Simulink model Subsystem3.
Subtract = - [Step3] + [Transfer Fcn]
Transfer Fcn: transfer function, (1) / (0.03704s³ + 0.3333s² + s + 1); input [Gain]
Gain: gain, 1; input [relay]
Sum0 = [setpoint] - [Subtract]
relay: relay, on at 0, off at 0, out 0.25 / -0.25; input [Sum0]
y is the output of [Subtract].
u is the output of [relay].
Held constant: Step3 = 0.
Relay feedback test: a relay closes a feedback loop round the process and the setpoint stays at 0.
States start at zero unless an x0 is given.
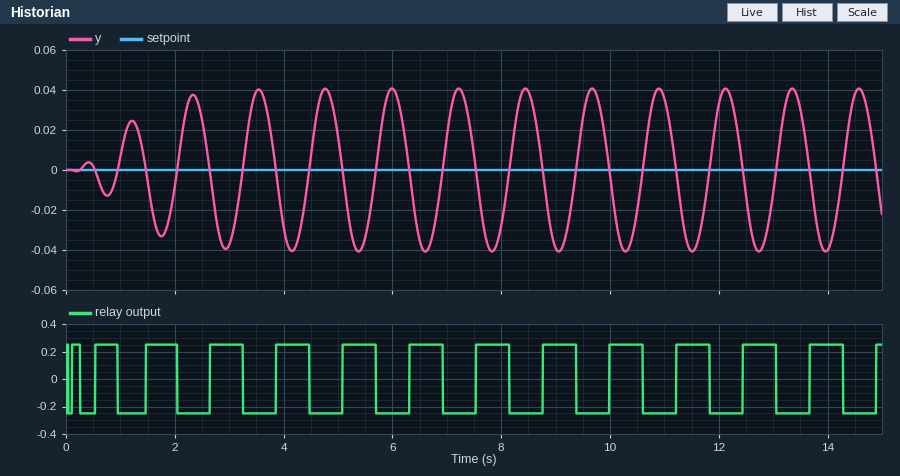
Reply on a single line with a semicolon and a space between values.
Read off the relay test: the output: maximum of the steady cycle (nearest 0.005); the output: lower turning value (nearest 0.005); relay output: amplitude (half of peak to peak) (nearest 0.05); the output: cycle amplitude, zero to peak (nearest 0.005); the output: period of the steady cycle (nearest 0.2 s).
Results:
0.040; -0.040; 0.25; 0.040; 1.2 s
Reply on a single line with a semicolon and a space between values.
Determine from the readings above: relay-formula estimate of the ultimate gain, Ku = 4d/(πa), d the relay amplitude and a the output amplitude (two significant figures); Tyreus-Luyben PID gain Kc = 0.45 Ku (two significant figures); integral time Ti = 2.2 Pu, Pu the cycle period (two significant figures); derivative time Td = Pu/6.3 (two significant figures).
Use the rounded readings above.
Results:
8.0; 3.6; 2.6 s; 0.19 s
